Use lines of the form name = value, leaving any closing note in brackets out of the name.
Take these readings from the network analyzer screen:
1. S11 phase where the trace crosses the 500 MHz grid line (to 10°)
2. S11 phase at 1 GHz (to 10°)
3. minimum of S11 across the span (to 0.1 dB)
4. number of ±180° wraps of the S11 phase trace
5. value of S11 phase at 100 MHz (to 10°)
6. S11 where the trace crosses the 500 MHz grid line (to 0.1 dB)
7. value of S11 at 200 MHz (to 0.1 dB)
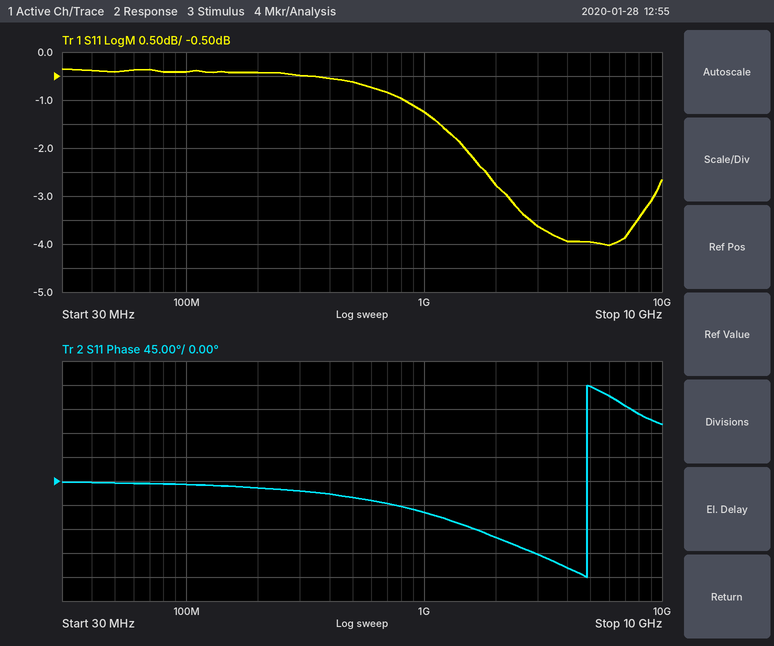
S11 phase where the trace crosses the 500 MHz grid line = -30°
S11 phase at 1 GHz = -60°
minimum of S11 across the span = -4.0 dB
number of ±180° wraps of the S11 phase trace = 1
value of S11 phase at 100 MHz = -10°
S11 where the trace crosses the 500 MHz grid line = -0.6 dB
value of S11 at 200 MHz = -0.4 dB
